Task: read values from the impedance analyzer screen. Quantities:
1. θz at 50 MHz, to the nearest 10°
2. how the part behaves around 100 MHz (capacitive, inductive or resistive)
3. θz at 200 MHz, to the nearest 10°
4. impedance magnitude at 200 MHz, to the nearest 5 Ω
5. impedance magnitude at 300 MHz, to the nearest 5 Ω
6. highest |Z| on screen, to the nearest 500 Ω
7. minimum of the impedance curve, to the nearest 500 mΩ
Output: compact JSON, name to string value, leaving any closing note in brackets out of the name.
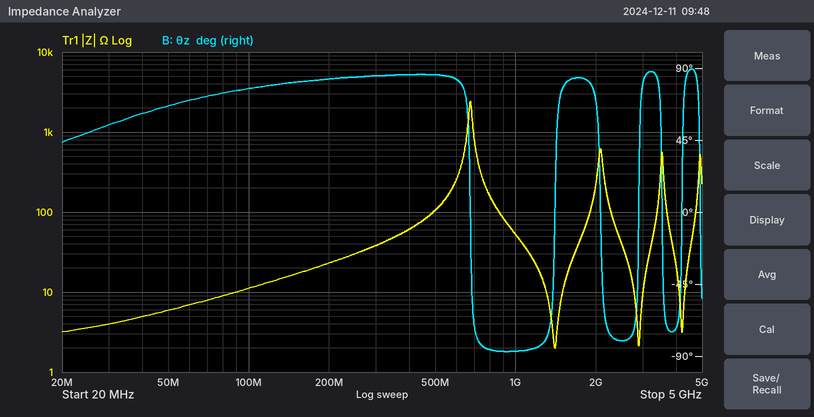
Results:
{"θz at 50 MHz, to the nearest 10°": "70°", "how the part behaves around 100 MHz": "inductive", "θz at 200 MHz, to the nearest 10°": "80°", "impedance magnitude at 200 MHz, to the nearest 5 Ω": "25 Ω", "impedance magnitude at 300 MHz, to the nearest 5 Ω": "40 Ω", "highest |Z| on screen, to the nearest 500 Ω": "2.5 kΩ", "minimum of the impedance curve, to the nearest 500 mΩ": "2.0 Ω"}
